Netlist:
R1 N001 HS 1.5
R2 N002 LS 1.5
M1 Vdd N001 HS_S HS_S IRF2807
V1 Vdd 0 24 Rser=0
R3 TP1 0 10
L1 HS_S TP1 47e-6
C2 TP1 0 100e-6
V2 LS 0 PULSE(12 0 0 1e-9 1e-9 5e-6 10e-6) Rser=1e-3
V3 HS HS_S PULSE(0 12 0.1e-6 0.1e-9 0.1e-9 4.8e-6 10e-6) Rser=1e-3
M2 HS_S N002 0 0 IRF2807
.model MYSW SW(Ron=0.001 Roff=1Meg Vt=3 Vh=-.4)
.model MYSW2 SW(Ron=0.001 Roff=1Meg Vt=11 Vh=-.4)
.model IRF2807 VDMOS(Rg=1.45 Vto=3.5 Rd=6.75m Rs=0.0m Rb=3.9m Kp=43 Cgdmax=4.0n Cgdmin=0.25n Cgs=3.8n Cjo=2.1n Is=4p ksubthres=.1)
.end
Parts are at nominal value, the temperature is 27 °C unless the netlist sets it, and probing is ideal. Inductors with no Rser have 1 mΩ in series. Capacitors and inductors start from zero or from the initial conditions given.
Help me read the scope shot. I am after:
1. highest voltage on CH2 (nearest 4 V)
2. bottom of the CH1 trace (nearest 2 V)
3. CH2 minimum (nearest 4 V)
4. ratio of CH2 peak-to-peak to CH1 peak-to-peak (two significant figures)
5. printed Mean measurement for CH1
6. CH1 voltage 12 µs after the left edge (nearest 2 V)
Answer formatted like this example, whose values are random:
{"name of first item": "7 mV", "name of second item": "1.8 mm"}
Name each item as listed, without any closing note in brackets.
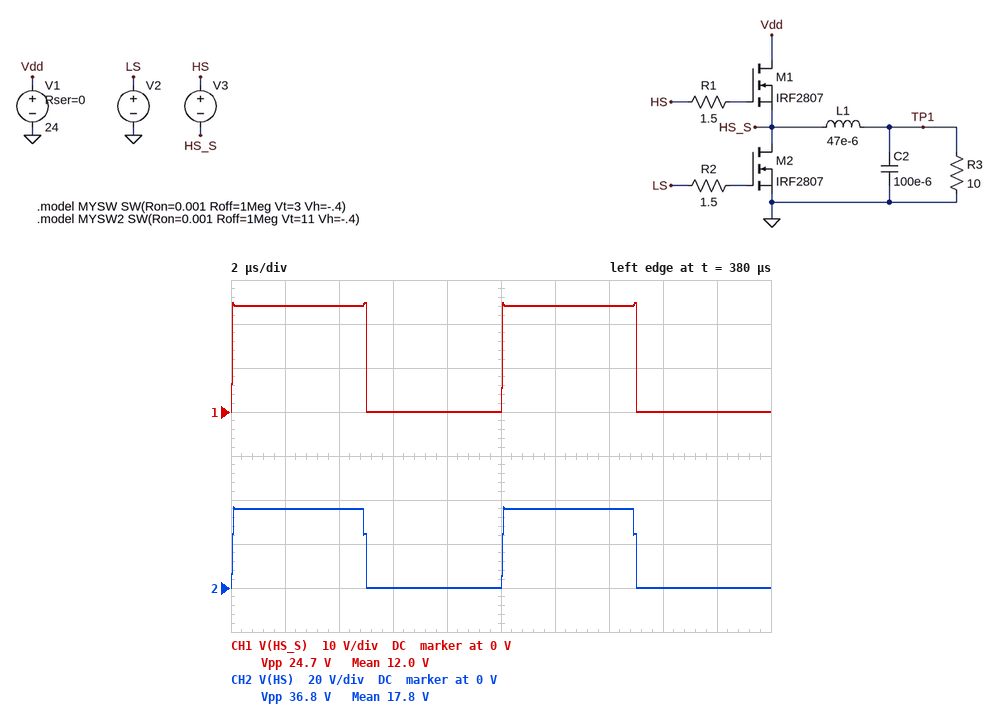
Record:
{"highest voltage on CH2": "36 V", "bottom of the CH1 trace": "0 V", "CH2 minimum": "0 V", "ratio of CH2 peak-to-peak to CH1 peak-to-peak": "1.5", "printed Mean measurement for CH1": "12.0 V", "CH1 voltage 12 µs after the left edge": "24 V"}
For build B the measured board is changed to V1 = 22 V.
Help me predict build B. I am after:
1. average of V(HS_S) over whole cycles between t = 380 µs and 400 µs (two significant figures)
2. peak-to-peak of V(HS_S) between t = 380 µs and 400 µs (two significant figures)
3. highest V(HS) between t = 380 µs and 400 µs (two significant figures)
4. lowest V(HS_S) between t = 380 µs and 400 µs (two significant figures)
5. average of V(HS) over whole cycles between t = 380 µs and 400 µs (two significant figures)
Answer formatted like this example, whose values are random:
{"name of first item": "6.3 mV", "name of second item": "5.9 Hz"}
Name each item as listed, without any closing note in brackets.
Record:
{"average of V(HS_S) over whole cycles between t = 380 µs and 400 µs": "11 V", "peak-to-peak of V(HS_S) between t = 380 µs and 400 µs": "23 V", "highest V(HS) between t = 380 µs and 400 µs": "35 V", "lowest V(HS_S) between t = 380 µs and 400 µs": "41 mV", "average of V(HS) over whole cycles between t = 380 µs and 400 µs": "17 V"}
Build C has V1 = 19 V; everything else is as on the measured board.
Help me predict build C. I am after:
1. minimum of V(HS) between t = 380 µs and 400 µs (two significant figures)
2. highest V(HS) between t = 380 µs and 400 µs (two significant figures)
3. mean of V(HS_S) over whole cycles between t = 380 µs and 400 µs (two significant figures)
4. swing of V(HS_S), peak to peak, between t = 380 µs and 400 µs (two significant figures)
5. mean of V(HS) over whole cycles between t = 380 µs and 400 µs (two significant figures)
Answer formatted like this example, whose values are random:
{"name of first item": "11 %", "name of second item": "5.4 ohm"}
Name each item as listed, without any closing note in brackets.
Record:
{"minimum of V(HS) between t = 380 µs and 400 µs": "34 mV", "highest V(HS) between t = 380 µs and 400 µs": "32 V", "mean of V(HS_S) over whole cycles between t = 380 µs and 400 µs": "9.5 V", "swing of V(HS_S), peak to peak, between t = 380 µs and 400 µs": "20 V", "mean of V(HS) over whole cycles between t = 380 µs and 400 µs": "15 V"}
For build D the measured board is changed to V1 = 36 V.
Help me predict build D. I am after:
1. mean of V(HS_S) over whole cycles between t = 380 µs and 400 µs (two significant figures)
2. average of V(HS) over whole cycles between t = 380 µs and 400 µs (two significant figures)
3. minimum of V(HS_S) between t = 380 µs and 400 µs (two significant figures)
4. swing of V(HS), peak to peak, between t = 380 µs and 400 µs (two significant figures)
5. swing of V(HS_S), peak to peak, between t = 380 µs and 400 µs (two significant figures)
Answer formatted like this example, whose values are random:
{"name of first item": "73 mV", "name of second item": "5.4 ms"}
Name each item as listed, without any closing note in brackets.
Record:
{"mean of V(HS_S) over whole cycles between t = 380 µs and 400 µs": "18 V", "average of V(HS) over whole cycles between t = 380 µs and 400 µs": "24 V", "minimum of V(HS_S) between t = 380 µs and 400 µs": "69 mV", "swing of V(HS), peak to peak, between t = 380 µs and 400 µs": "49 V", "swing of V(HS_S), peak to peak, between t = 380 µs and 400 µs": "37 V"}
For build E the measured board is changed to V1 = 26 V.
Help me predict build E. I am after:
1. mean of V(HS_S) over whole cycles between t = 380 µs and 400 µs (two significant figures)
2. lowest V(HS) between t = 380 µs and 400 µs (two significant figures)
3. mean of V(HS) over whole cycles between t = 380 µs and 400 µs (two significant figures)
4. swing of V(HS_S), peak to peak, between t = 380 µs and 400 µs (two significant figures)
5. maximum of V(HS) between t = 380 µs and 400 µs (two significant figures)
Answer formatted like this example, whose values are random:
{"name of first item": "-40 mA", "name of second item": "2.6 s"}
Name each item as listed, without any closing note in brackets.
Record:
{"mean of V(HS_S) over whole cycles between t = 380 µs and 400 µs": "13 V", "lowest V(HS) between t = 380 µs and 400 µs": "49 mV", "mean of V(HS) over whole cycles between t = 380 µs and 400 µs": "19 V", "swing of V(HS_S), peak to peak, between t = 380 µs and 400 µs": "27 V", "maximum of V(HS) between t = 380 µs and 400 µs": "39 V"}
